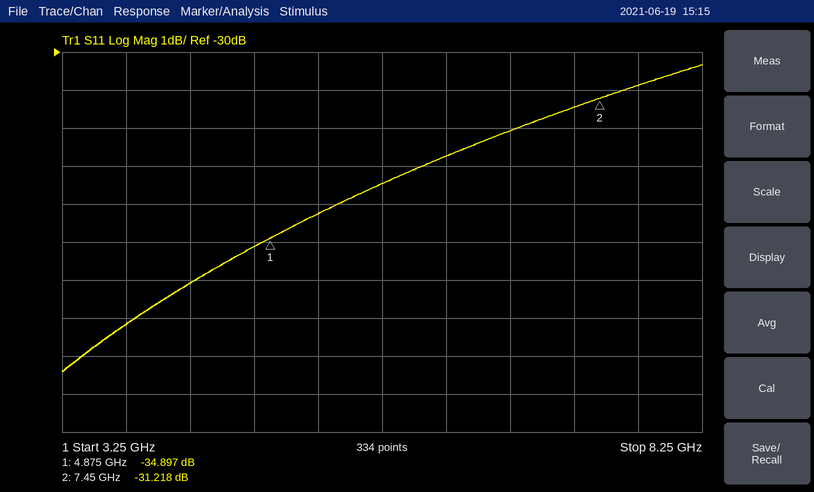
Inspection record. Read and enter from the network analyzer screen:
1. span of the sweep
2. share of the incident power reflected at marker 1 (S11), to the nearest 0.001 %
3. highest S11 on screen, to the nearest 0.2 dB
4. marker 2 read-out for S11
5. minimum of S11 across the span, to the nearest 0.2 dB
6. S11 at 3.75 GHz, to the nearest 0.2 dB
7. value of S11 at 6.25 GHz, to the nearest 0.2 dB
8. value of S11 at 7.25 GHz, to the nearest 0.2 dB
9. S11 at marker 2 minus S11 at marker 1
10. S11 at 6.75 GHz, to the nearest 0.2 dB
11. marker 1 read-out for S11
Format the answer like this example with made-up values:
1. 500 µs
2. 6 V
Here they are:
1. 5 GHz
2. 0.032 %
3. -30.4 dB
4. -31.218 dB
5. -38.4 dB
6. -37.2 dB
7. -32.8 dB
8. -31.4 dB
9. 3.679 dB
10. -32.0 dB
11. -34.897 dB
